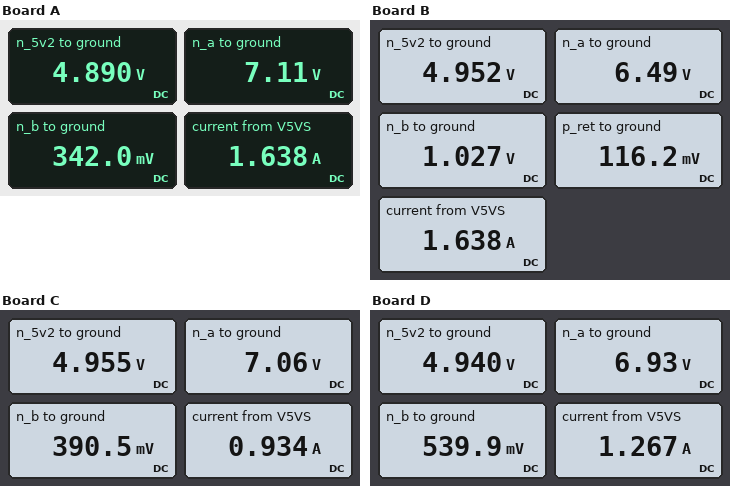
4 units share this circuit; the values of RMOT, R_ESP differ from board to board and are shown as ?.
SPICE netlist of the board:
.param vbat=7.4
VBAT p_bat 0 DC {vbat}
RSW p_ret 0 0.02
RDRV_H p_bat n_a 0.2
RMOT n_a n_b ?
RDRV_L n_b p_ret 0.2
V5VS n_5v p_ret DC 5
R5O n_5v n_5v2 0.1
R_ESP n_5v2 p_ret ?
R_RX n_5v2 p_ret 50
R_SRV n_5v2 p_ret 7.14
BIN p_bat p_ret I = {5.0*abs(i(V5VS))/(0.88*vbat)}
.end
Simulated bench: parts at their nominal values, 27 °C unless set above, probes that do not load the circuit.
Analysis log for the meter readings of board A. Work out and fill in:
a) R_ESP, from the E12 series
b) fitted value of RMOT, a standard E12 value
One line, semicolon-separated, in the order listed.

5.6 Ω; 4.7 Ω
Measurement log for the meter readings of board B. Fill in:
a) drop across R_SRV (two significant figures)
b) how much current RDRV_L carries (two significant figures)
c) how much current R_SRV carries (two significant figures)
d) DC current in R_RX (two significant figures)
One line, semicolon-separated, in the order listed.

4.8 V; 4.6 A; 680 mA; 97 mA
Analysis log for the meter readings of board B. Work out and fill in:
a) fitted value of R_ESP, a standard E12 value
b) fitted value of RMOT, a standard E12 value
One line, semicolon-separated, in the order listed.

5.6 Ω; 1.2 Ω
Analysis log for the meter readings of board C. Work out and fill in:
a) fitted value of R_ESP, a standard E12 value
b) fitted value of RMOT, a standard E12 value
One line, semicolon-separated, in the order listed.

33 Ω; 3.9 Ω
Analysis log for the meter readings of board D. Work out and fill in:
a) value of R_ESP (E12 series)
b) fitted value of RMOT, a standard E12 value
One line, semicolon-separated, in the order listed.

10 Ω; 2.7 Ω
